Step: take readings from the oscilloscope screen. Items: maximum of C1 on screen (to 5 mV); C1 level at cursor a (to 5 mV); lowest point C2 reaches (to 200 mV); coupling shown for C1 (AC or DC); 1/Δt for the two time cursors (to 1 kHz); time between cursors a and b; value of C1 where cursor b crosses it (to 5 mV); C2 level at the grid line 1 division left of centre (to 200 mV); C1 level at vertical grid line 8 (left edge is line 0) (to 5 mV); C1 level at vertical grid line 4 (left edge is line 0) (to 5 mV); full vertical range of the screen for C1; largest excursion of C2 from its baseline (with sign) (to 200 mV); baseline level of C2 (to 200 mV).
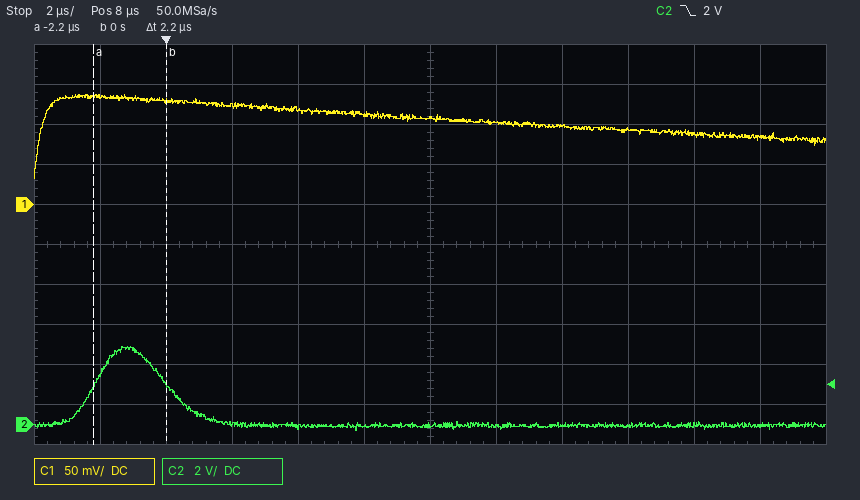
140 mV
135 mV
-400 mV
DC
455 kHz
2.2 µs
130 mV
0.0 V
100 mV
120 mV
500 mV
+4.0 V
0.0 V
